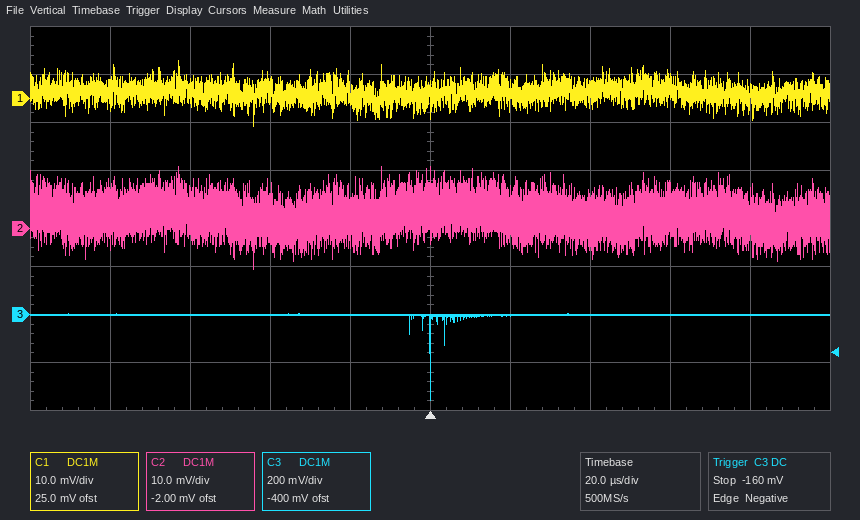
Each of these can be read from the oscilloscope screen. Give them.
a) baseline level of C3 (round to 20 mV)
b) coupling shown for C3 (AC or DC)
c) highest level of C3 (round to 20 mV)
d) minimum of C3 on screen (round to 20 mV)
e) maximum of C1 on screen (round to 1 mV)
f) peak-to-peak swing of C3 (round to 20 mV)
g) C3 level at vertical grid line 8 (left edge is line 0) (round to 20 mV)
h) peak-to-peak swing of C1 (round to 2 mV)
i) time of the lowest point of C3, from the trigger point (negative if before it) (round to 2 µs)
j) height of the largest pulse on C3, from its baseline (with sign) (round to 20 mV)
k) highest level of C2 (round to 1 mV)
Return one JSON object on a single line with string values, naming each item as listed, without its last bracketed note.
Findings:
{"baseline level of C3": "0 mV", "coupling shown for C3": "DC", "highest level of C3": "0 mV", "minimum of C3 on screen": "-360 mV", "maximum of C1 on screen": "8 mV", "peak-to-peak swing of C3": "360 mV", "C3 level at vertical grid line 8 (left edge is line 0)": "0 mV", "peak-to-peak swing of C1": "14 mV", "time of the lowest point of C3, from the trigger point (negative if before it)": "0 µs", "height of the largest pulse on C3, from its baseline (with sign)": "-360 mV", "highest level of C2": "13 mV"}
